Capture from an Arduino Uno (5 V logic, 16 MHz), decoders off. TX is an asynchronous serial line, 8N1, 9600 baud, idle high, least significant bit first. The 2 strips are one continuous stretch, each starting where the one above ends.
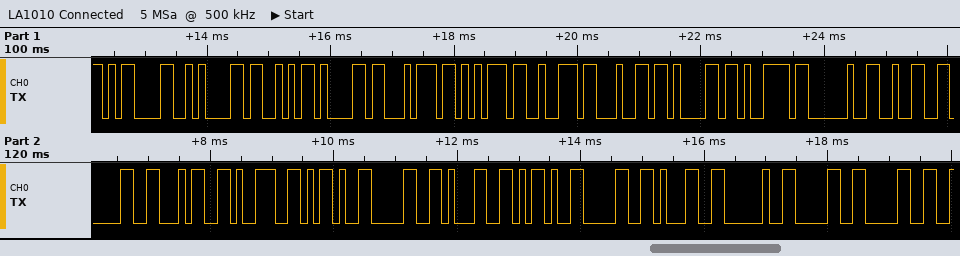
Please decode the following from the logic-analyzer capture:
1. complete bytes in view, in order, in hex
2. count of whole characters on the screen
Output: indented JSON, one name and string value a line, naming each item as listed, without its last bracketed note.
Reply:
{
  "complete bytes in view, in order, in hex": "0x0D 0x0A 0x53 0x61 0x74 0x75 0x72 0x64 0x61 0x79 0x20 0x32 0x30 0x34 0x39 0x2D 0x30 0x31 0x2D 0x30 0x31 0x20 0x30 0x30",
  "count of whole characters on the screen": "24"
}
